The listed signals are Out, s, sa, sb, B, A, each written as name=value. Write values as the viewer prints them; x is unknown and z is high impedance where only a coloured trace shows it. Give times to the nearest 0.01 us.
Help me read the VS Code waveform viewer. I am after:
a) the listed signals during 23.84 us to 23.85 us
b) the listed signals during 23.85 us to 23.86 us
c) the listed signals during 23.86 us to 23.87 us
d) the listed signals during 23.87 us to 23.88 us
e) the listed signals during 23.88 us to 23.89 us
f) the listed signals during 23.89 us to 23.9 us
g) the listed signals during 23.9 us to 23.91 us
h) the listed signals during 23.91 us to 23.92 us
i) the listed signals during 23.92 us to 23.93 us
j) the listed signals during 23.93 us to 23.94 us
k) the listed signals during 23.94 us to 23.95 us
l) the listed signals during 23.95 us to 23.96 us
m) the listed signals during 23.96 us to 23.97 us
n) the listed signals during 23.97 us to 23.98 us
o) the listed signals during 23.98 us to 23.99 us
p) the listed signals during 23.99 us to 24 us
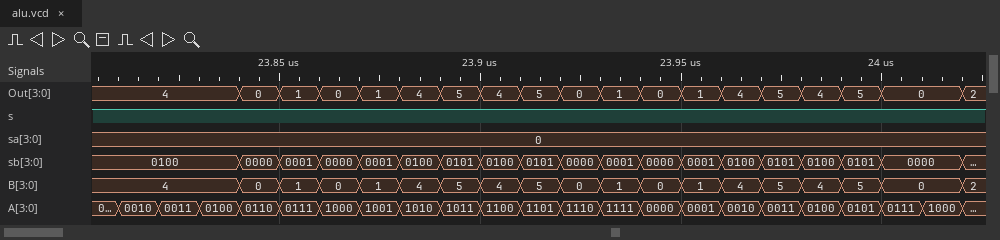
Out=0, s=1, sa=0, sb=0000, B=0, A=0110
Out=1, s=1, sa=0, sb=0001, B=1, A=0111
Out=0, s=1, sa=0, sb=0000, B=0, A=1000
Out=1, s=1, sa=0, sb=0001, B=1, A=1001
Out=4, s=1, sa=0, sb=0100, B=4, A=1010
Out=5, s=1, sa=0, sb=0101, B=5, A=1011
Out=4, s=1, sa=0, sb=0100, B=4, A=1100
Out=5, s=1, sa=0, sb=0101, B=5, A=1101
Out=0, s=1, sa=0, sb=0000, B=0, A=1110
Out=1, s=1, sa=0, sb=0001, B=1, A=1111
Out=0, s=1, sa=0, sb=0000, B=0, A=0000
Out=1, s=1, sa=0, sb=0001, B=1, A=0001
Out=4, s=1, sa=0, sb=0100, B=4, A=0010
Out=5, s=1, sa=0, sb=0101, B=5, A=0011
Out=4, s=1, sa=0, sb=0100, B=4, A=0100
Out=5, s=1, sa=0, sb=0101, B=5, A=0101
